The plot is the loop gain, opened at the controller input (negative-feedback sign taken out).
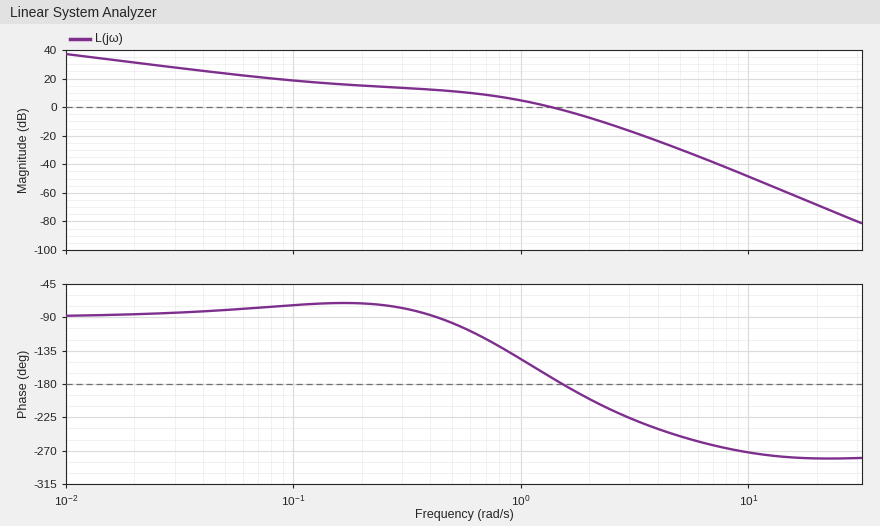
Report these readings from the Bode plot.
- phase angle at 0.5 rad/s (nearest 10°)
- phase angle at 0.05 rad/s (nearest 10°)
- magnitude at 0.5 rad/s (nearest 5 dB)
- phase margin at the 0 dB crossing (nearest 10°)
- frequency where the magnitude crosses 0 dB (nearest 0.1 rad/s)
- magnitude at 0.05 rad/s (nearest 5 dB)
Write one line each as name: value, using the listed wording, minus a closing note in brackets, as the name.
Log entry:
phase angle at 0.5 rad/s: -100°
phase angle at 0.05 rad/s: -80°
magnitude at 0.5 rad/s: 10 dB
phase margin at the 0 dB crossing: 10°
frequency where the magnitude crosses 0 dB: 1.4 rad/s
magnitude at 0.05 rad/s: 25 dB
